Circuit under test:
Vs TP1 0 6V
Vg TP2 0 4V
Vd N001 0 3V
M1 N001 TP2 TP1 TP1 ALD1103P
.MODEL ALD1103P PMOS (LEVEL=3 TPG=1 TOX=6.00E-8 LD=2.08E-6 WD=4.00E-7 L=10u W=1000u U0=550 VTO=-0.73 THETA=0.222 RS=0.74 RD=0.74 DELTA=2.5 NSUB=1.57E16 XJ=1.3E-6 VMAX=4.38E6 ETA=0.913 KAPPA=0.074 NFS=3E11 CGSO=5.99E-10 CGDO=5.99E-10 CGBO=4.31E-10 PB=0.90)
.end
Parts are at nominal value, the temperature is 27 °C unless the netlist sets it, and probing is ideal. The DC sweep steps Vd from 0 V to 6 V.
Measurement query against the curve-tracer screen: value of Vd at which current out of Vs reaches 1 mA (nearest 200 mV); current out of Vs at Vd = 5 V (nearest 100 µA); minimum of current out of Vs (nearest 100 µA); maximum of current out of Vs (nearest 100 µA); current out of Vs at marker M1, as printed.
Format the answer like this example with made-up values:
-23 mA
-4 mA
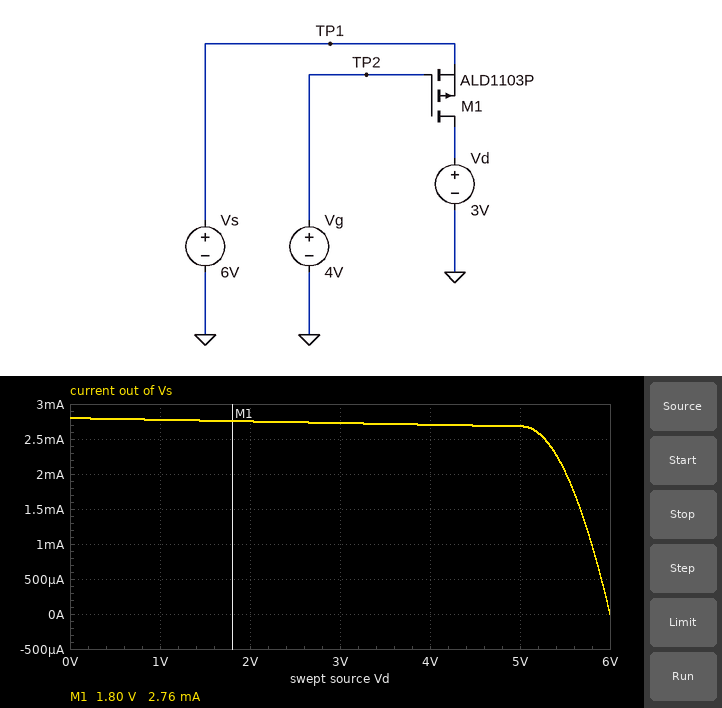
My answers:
5.8 V
2.7 mA
0 A
2.8 mA
2.76 mA
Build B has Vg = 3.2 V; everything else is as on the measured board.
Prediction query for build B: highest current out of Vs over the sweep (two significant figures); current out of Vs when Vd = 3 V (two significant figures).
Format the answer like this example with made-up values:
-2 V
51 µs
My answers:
6.2 mA
6.1 mA
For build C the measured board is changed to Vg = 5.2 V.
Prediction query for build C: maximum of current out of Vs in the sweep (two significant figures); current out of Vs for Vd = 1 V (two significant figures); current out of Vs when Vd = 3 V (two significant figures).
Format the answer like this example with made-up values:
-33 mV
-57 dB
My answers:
45 µA
42 µA
35 µA
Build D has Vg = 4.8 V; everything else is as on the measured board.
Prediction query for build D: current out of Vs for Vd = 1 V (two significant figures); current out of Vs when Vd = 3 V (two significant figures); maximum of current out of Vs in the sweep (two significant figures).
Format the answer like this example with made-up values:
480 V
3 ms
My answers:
530 µA
510 µA
540 µA
